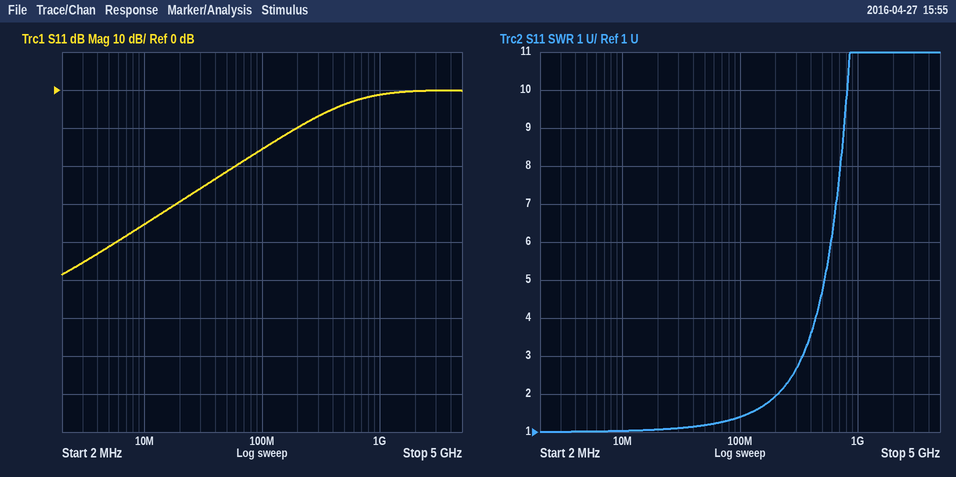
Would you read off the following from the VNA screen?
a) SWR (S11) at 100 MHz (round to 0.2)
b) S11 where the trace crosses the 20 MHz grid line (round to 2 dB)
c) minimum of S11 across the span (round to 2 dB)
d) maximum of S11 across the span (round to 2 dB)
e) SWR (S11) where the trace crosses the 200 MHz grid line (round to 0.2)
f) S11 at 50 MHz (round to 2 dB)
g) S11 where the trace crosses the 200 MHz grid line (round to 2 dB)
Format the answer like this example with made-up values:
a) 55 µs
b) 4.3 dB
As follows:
a) 1.4
b) -30 dB
c) -48 dB
d) 0 dB
e) 2.0
f) -22 dB
g) -10 dB
